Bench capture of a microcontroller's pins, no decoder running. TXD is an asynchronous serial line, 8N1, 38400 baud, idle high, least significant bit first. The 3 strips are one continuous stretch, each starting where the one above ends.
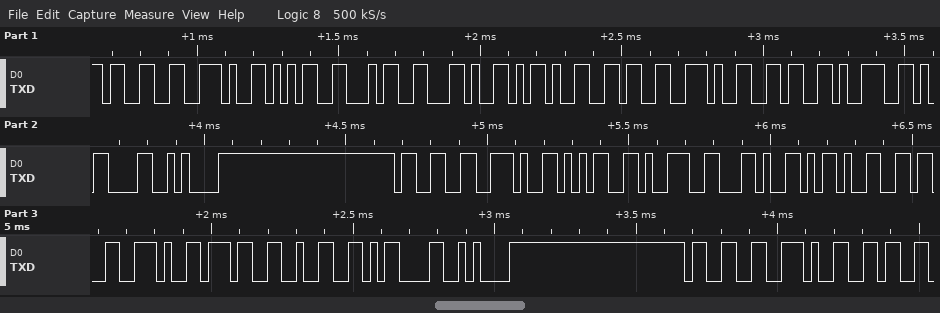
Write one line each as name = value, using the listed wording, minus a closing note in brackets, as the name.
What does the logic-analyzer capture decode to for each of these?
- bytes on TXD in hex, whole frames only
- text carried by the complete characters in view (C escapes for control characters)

bytes on TXD in hex, whole frames only = 33 2E 35 34 2C 2D 36 2E 36 39 0D 0A 33 2E 35 39 2C 2D 36 2E 37 32 0D 0A 33 2E 36
text carried by the complete characters in view = "3.54,-6.69\r\n3.59,-6.72\r\n3.6"
